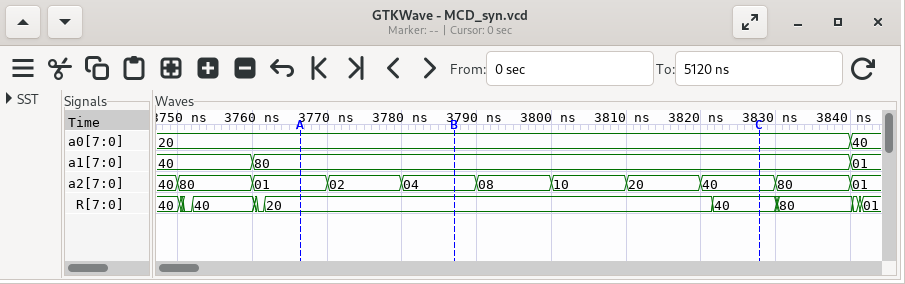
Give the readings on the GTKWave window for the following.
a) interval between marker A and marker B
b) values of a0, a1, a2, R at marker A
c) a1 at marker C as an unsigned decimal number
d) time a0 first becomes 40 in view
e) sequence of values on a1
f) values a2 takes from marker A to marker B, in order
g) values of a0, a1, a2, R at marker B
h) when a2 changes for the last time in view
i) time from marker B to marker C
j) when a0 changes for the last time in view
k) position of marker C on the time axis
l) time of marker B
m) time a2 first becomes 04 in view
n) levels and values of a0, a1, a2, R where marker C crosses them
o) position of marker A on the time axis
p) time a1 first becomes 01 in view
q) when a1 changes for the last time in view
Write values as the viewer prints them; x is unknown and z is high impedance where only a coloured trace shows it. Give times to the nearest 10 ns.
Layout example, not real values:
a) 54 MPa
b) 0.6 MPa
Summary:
a) 20 ns
b) a0=20, a1=80, a2=01, R=20
c) 128
d) 3840 ns
e) 40, 80, 01
f) 01, 02, 04
g) a0=20, a1=80, a2=04, R=20
h) 3840 ns
i) 40 ns
j) 3840 ns
k) 3830 ns
l) 3790 ns
m) 3780 ns
n) a0=20, a1=80, a2=40, R=40
o) 3770 ns
p) 3840 ns
q) 3840 ns
